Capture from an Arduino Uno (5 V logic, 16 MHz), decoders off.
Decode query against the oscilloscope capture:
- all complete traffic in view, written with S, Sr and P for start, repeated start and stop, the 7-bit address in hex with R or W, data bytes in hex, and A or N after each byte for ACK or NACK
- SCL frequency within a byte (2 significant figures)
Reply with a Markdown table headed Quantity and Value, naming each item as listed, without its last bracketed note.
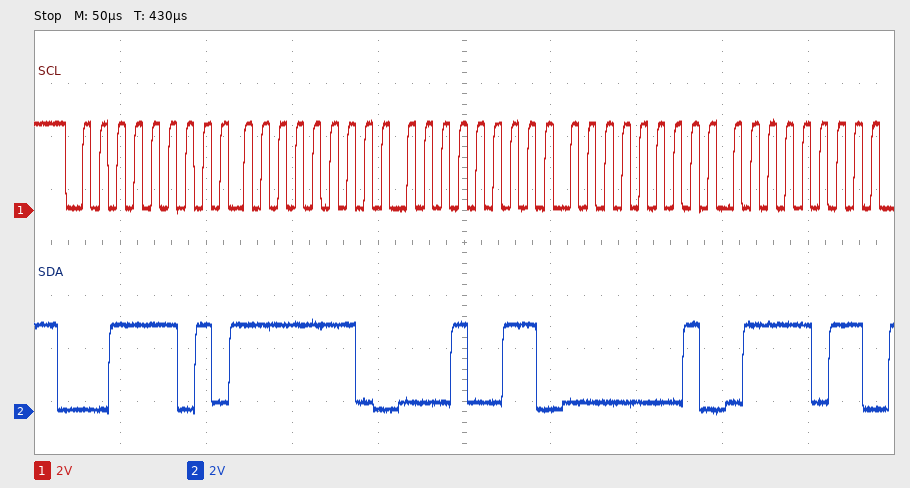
| Quantity | Value |
|---|---|
| all complete traffic in view, written with S, Sr and P for start, repeated start and stop, the 7-bit address in hex with R or W, data bytes in hex, and A or N after each byte for ACK or NACK | S 1ER A FE A 13 A 01 A 7B A |
| SCL frequency within a byte | 100 kHz |
